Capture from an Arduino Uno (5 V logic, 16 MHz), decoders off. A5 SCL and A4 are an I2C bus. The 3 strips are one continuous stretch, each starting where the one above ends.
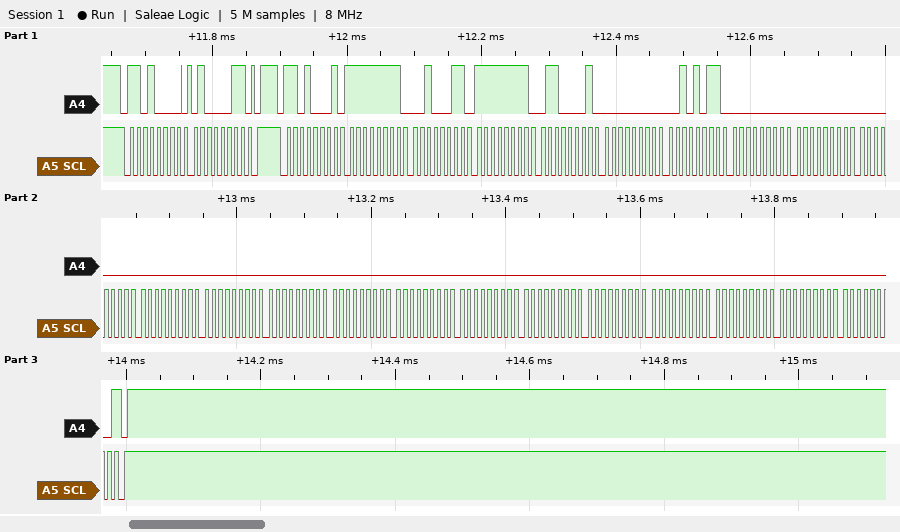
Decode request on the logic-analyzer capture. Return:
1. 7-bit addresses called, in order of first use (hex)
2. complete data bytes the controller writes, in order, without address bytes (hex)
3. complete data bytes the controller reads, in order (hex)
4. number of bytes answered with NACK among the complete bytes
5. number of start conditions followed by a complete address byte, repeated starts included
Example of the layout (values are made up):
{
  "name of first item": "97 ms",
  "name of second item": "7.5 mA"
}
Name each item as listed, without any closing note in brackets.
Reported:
{
  "7-bit addresses called, in order of first use": "0x68",
  "complete data bytes the controller writes, in order, without address bytes": "43",
  "complete data bytes the controller reads, in order": "FF 23 FF 61 00 2B 00 00 00 00 00 00 00 00 00 00 00 00 00 00 00",
  "number of bytes answered with NACK among the complete bytes": "1",
  "number of start conditions followed by a complete address byte, repeated starts included": "2"
}
